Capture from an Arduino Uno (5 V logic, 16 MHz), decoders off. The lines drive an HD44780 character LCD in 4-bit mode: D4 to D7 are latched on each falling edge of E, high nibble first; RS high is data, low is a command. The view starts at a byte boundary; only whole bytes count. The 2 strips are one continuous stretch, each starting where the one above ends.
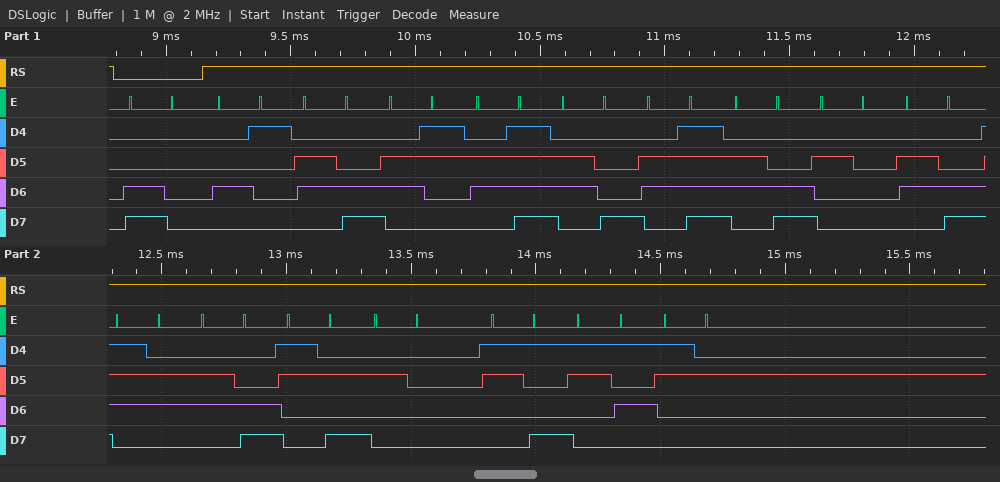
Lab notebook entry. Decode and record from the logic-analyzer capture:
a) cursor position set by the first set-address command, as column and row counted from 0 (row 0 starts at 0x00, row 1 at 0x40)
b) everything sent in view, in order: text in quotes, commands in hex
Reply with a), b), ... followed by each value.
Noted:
a) column 0, row 1
b) 0xC0 "Alcohol lvl: 952"
